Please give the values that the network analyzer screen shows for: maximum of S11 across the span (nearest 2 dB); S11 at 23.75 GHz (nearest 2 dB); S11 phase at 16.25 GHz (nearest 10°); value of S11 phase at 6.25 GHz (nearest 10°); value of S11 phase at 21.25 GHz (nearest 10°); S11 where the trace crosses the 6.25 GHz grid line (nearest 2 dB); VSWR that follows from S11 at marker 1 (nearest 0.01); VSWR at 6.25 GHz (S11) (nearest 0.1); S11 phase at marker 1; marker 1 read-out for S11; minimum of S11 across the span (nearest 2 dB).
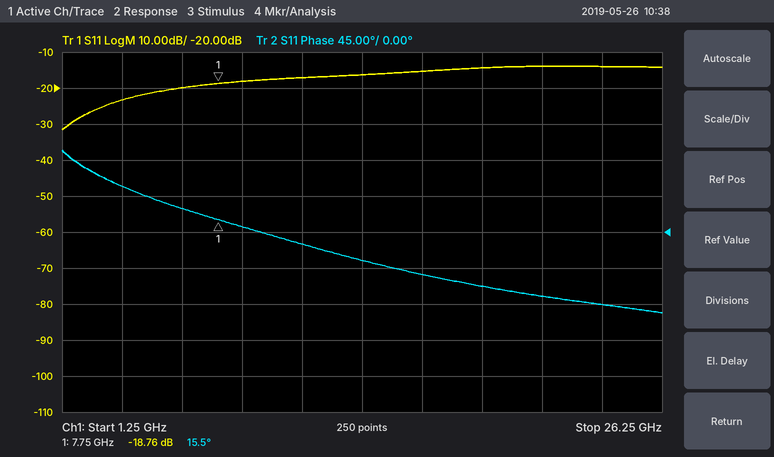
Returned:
-14 dB
-14 dB
-50°
30°
-80°
-20 dB
1.26
1.2
15.5°
-18.76 dB
-32 dB
